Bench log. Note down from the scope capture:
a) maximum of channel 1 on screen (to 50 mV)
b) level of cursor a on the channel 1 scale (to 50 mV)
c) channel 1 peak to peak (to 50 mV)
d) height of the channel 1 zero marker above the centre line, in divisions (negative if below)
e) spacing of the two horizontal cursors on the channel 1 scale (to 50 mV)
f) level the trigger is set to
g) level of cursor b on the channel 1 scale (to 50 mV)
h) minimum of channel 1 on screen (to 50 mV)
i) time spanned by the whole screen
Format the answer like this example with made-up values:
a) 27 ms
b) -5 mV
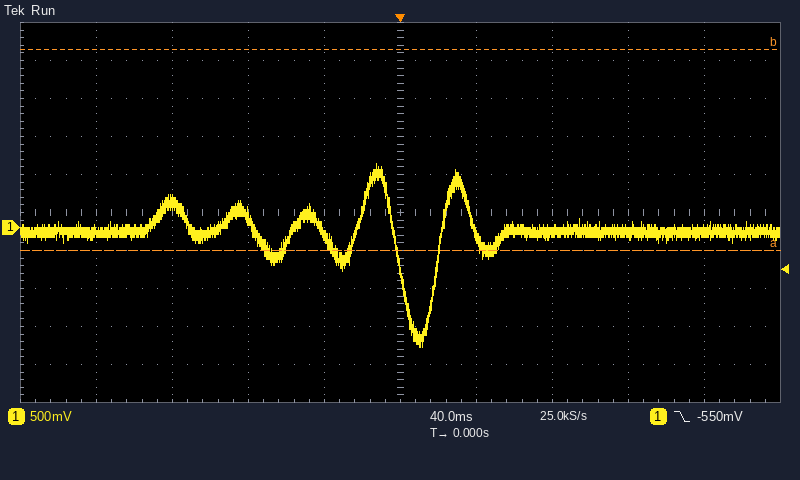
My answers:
a) 850 mV
b) -300 mV
c) 2.40 V
d) -0.4 div
e) 2.65 V
f) -550 mV
g) 2.35 V
h) -1.55 V
i) 400 ms
